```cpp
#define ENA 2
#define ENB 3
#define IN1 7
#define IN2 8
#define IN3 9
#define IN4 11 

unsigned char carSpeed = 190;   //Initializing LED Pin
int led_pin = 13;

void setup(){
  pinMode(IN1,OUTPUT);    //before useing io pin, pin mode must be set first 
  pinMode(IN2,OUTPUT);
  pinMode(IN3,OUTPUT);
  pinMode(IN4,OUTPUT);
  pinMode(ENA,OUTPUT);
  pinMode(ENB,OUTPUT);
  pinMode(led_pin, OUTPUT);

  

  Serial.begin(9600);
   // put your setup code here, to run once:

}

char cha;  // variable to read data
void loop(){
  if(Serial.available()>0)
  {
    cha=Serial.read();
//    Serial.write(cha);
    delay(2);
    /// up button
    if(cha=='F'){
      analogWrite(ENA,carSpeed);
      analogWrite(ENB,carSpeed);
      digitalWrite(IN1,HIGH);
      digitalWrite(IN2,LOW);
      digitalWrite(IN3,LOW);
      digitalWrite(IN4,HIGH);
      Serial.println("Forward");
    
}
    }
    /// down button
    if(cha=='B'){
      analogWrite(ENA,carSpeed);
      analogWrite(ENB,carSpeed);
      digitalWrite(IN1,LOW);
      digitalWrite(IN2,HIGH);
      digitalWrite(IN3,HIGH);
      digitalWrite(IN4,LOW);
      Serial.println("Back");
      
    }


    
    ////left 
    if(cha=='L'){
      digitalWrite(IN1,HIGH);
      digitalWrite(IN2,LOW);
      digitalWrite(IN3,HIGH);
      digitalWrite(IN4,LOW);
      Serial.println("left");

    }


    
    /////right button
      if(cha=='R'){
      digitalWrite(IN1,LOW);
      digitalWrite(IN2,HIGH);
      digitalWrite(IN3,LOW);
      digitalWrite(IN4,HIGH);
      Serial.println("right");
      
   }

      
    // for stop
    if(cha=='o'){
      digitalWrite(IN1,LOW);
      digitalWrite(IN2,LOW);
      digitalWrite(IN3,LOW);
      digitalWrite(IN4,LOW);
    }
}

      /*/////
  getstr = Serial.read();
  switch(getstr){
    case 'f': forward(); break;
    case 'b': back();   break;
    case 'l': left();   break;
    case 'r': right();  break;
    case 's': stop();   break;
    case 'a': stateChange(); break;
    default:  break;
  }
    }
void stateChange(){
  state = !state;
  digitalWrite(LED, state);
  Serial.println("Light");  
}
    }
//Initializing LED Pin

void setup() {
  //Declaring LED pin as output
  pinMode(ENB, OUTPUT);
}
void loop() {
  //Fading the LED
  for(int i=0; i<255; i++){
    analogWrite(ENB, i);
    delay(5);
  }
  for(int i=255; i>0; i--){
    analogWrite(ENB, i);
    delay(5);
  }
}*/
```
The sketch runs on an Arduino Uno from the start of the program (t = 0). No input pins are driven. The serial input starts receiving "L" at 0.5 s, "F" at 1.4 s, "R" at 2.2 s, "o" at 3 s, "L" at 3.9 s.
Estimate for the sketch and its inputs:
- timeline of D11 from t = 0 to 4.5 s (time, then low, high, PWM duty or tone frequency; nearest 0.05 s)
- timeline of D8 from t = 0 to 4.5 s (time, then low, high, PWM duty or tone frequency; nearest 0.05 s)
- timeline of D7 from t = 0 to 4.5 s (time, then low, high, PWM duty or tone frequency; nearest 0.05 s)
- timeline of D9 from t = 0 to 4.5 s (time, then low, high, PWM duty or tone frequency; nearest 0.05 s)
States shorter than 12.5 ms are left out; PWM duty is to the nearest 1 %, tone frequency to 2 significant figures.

0 s low; 1.4 s high; 3 s low
0 s low; 2.2 s high; 3 s low
0 s low; 0.5 s high; 2.2 s low; 3.9 s high
0 s low; 0.5 s high; 1.4 s low; 3.9 s high
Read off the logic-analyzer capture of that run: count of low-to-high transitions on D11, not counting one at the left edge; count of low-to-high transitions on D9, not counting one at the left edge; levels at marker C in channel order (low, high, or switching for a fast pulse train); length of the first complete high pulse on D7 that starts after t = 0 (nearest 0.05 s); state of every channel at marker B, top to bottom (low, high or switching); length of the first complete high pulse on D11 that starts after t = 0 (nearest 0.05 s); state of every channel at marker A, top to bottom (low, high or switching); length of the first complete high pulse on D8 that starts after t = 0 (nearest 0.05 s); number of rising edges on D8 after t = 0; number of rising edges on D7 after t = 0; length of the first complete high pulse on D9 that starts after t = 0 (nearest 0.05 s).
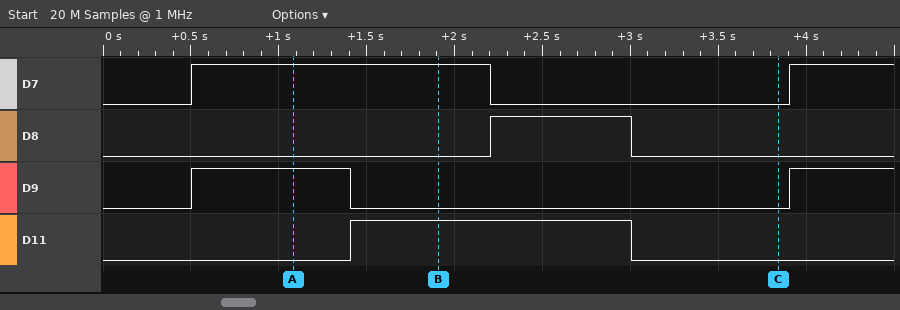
1
2
D7 low, D8 low, D9 low, D11 low
1.70 s
D7 high, D8 low, D9 low, D11 high
1.60 s
D7 high, D8 low, D9 high, D11 low
0.80 s
1
2
0.90 s
